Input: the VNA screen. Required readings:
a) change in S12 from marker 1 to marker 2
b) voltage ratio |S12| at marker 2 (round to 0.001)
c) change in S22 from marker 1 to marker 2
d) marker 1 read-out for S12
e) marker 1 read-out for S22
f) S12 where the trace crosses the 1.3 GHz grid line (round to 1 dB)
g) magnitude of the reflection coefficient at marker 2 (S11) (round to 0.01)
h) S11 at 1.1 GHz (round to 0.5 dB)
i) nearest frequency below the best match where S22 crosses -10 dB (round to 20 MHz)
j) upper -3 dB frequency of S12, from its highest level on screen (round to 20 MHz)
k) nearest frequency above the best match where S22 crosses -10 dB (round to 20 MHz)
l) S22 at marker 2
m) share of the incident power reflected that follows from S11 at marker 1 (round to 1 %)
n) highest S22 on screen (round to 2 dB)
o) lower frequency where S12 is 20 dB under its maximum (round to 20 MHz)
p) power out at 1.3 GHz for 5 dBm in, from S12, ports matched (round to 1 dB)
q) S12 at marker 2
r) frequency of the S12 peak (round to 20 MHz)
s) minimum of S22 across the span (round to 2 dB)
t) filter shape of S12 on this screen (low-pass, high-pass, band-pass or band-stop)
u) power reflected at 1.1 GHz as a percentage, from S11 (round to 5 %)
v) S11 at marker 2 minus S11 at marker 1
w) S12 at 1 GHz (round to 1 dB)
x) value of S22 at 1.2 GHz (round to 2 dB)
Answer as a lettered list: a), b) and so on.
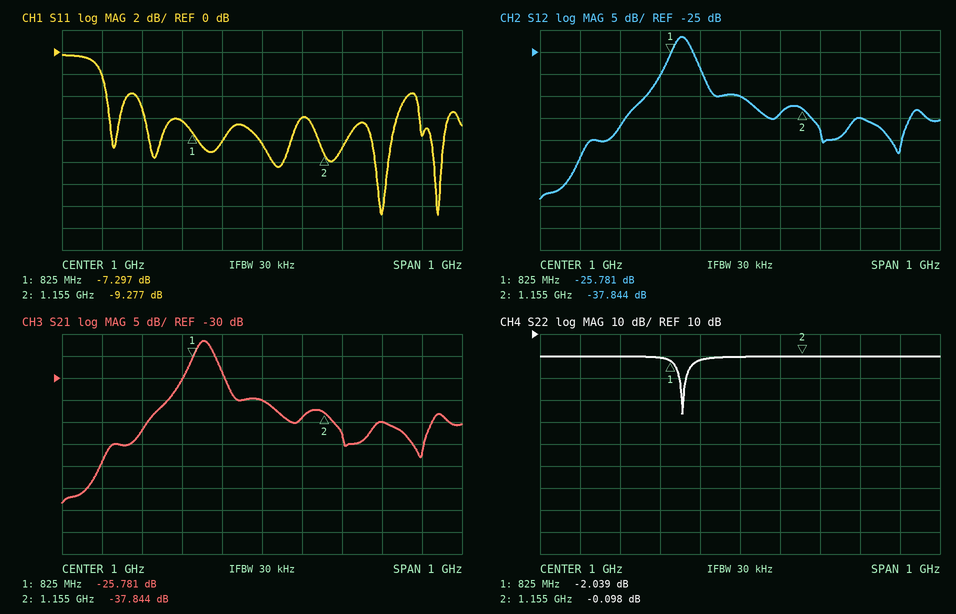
a) -12.063 dB
b) 0.013
c) 1.941 dB
d) -25.781 dB
e) -2.039 dB
f) -40 dB
g) 0.34
h) -6.0 dB
i) 840 MHz
j) 880 MHz
k) 860 MHz
l) -0.098 dB
m) 19 %
n) 0 dB
o) 700 MHz
p) -35 dBm
q) -37.844 dB
r) 860 MHz
s) -26 dB
t) band-pass
u) 25 %
v) -1.980 dB
w) -35 dB
x) 0 dB
